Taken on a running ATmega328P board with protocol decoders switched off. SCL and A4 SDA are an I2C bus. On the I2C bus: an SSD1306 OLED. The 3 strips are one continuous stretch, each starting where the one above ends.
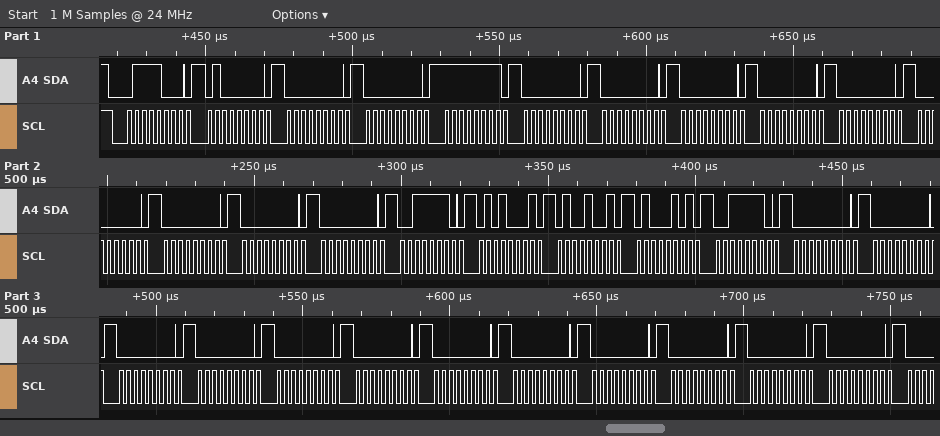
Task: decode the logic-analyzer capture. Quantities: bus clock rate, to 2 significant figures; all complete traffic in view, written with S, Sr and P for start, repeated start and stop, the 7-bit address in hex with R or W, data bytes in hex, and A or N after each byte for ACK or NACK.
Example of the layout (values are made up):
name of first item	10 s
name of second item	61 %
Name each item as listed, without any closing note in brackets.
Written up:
bus clock rate, to 2 significant figures	400 kHz
all complete traffic in view, written with S, Sr and P for start, repeated start and stop, the 7-bit address in hex with R or W, data bytes in hex, and A or N after each byte for ACK or NACK	S 3CW A 40 A 00 A 00 A FF A 00 A 00 A 00 A 00 A 00 A 00 A 00 A 00 A 00 A 3E A 51 A 49 A 45 A 3E A 00 A 00 A 00 A 00 A 00 A 00 A 00 A 00 A 00 A 00 A 00 A 00 A
